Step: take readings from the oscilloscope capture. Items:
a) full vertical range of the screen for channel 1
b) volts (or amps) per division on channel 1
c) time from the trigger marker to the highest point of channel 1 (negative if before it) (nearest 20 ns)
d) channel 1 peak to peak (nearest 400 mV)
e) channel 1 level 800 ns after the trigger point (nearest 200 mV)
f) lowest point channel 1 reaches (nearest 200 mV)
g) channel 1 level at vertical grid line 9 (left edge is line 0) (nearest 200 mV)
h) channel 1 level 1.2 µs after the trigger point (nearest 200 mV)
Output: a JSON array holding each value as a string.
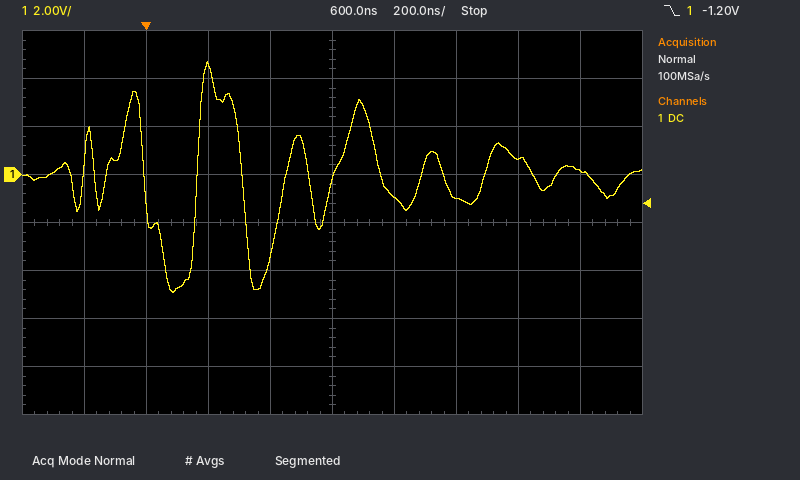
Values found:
["16 V", "2 V", "+200 ns", "9.6 V", "-1.0 V", "-5.0 V", "200 mV", "600 mV"]
